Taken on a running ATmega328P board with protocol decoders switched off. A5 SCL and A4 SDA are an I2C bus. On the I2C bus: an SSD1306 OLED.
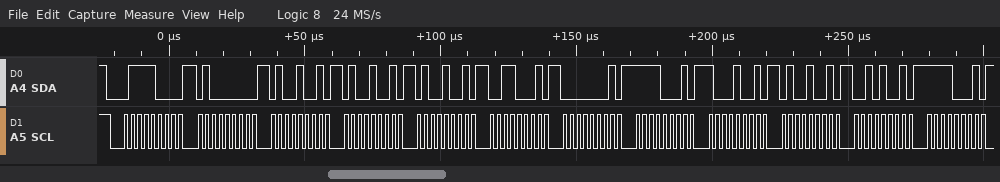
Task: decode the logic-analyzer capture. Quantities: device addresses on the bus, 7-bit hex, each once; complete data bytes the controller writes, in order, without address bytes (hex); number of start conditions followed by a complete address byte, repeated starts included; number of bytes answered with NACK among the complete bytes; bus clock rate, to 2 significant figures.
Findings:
0x3C
40 49 49 49 31 01 F1 89 49 29 F1
1
0
400 kHz
